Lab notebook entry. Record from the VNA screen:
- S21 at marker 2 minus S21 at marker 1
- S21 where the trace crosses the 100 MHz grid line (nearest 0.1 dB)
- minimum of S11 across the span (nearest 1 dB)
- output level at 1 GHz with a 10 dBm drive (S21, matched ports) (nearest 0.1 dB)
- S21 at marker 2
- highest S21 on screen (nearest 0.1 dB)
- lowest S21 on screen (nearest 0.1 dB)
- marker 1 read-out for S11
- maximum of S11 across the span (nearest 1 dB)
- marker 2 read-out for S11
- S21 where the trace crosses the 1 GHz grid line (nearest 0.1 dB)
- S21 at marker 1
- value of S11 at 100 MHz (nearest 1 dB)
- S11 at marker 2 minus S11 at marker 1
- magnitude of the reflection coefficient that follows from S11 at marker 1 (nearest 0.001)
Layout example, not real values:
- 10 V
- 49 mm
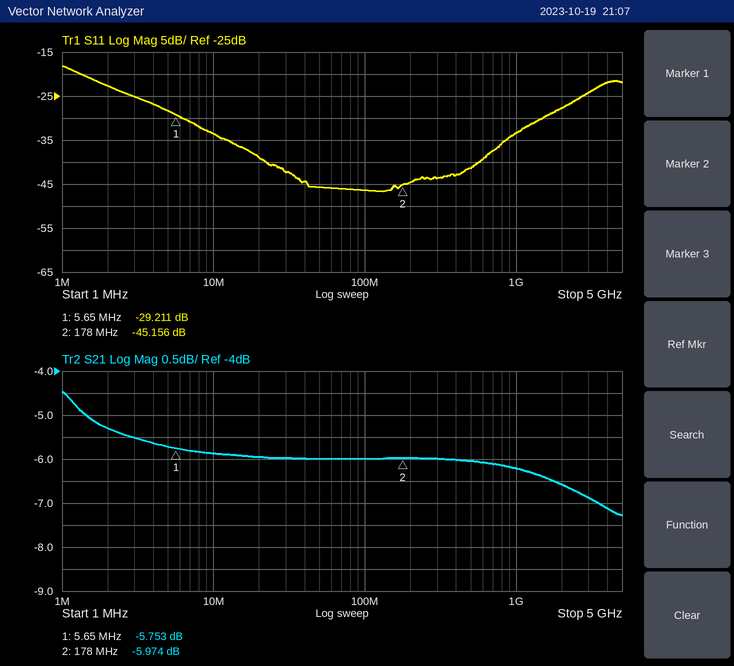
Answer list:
- -0.221 dB
- -6.0 dB
- -47 dB
- 3.8 dBm
- -5.974 dB
- -4.5 dB
- -7.3 dB
- -29.211 dB
- -18 dB
- -45.156 dB
- -6.2 dB
- -5.753 dB
- -46 dB
- -15.945 dB
- 0.035
